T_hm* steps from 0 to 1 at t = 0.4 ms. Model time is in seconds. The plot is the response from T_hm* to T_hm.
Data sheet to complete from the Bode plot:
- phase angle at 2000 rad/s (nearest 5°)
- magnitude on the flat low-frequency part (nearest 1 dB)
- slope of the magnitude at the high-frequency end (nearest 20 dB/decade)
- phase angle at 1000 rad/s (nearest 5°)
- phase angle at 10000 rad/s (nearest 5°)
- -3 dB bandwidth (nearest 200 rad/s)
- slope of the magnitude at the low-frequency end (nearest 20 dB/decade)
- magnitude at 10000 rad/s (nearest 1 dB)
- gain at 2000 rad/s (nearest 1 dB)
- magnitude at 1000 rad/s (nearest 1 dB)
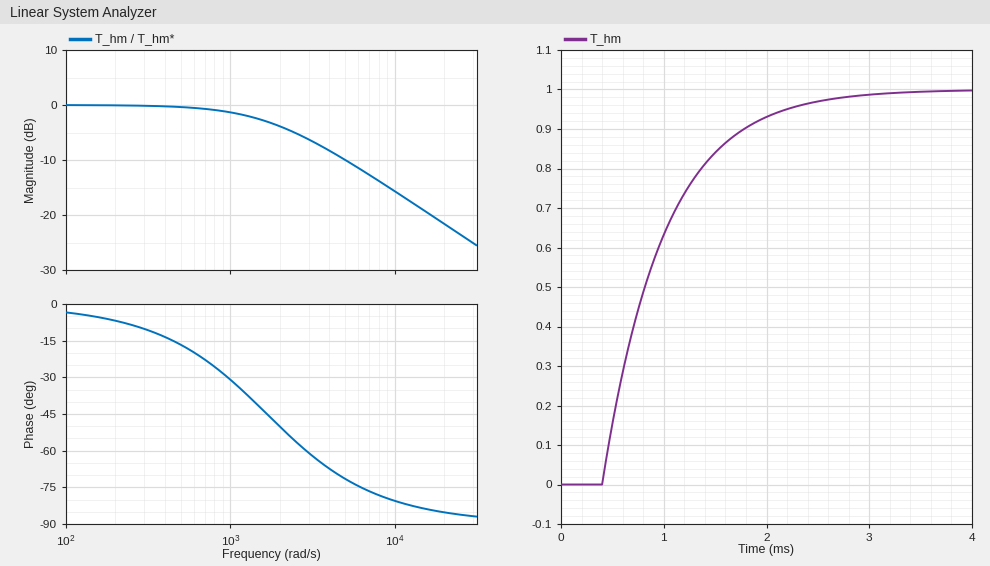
-50°
0 dB
-20 dB/decade
-30°
-80°
1600 rad/s
0 dB/decade
-16 dB
-4 dB
-1 dB
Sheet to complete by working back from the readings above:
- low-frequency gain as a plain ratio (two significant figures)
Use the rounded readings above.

1.0
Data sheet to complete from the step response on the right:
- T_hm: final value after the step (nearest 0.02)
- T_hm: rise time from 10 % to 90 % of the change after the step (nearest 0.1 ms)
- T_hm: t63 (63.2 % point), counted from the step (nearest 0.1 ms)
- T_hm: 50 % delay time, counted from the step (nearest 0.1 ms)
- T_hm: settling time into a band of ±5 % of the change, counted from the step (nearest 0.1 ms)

1.00
1.3 ms
0.6 ms
0.4 ms
1.8 ms
